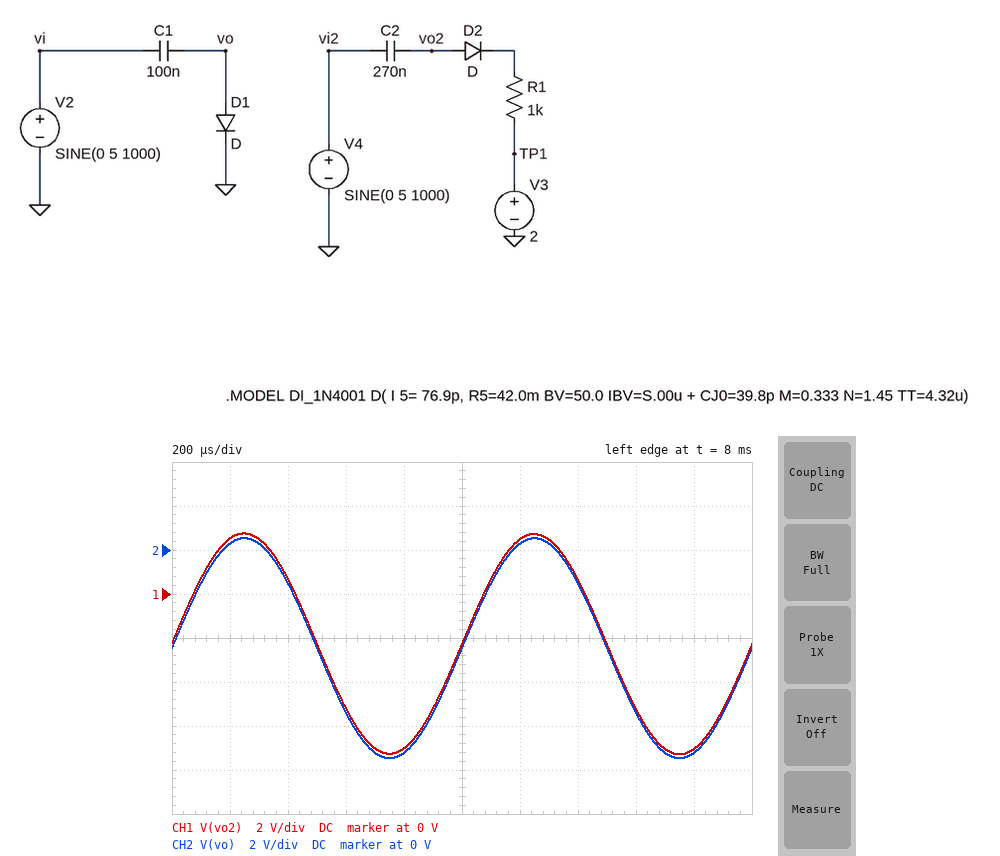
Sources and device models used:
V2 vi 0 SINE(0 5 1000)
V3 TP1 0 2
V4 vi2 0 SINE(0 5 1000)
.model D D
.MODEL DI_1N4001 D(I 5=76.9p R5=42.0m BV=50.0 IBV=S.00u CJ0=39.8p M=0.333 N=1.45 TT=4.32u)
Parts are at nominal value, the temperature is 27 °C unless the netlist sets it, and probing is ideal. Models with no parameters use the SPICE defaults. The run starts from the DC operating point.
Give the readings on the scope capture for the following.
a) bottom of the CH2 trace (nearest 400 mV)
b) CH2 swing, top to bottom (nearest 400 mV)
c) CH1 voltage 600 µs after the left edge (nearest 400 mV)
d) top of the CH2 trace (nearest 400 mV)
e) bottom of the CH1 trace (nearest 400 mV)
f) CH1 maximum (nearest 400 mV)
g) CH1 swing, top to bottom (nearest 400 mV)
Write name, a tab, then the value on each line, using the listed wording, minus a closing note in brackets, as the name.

bottom of the CH2 trace	-9.6 V
CH2 swing, top to bottom	10.0 V
CH1 voltage 600 µs after the left edge	-5.2 V
top of the CH2 trace	400 mV
bottom of the CH1 trace	-7.2 V
CH1 maximum	2.8 V
CH1 swing, top to bottom	10.0 V
